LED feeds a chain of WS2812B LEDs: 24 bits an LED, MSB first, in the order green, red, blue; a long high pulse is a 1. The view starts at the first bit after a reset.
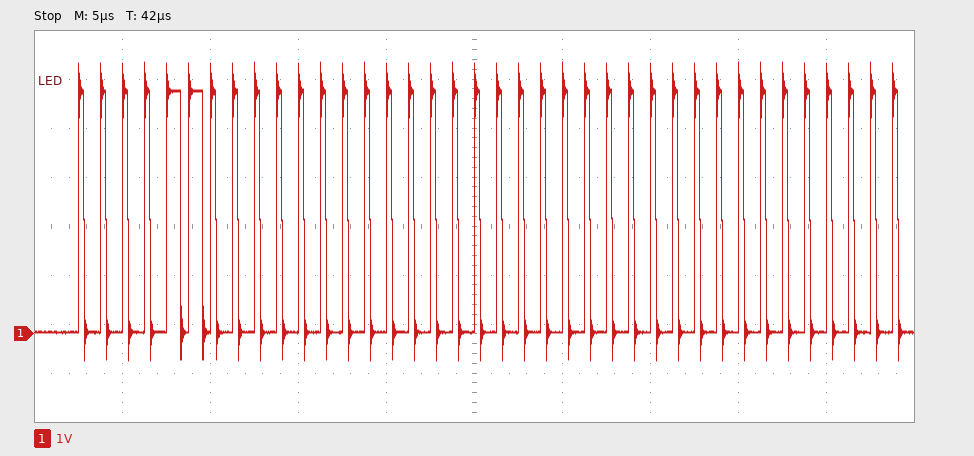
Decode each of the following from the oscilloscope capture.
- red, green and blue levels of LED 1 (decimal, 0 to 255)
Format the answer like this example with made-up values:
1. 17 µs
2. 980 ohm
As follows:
1. 0, 12, 0
